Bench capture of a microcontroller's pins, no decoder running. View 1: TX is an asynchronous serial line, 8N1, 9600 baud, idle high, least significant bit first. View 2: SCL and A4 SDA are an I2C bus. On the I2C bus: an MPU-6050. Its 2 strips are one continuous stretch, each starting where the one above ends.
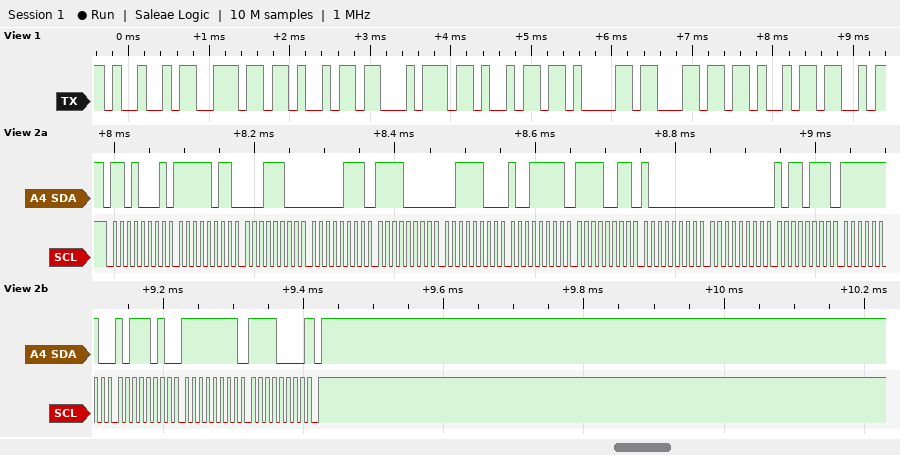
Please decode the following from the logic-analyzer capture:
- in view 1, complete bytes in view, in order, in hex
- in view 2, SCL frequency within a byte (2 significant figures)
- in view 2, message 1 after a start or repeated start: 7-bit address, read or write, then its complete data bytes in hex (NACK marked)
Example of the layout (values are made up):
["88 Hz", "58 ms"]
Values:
["49 6E 69 74 69 61 6C 69", "100 kHz", "0x68 read: FB 1C 07 F0 3C 9F F3 80 00 B7 FE BA FF F0 NACK"]
